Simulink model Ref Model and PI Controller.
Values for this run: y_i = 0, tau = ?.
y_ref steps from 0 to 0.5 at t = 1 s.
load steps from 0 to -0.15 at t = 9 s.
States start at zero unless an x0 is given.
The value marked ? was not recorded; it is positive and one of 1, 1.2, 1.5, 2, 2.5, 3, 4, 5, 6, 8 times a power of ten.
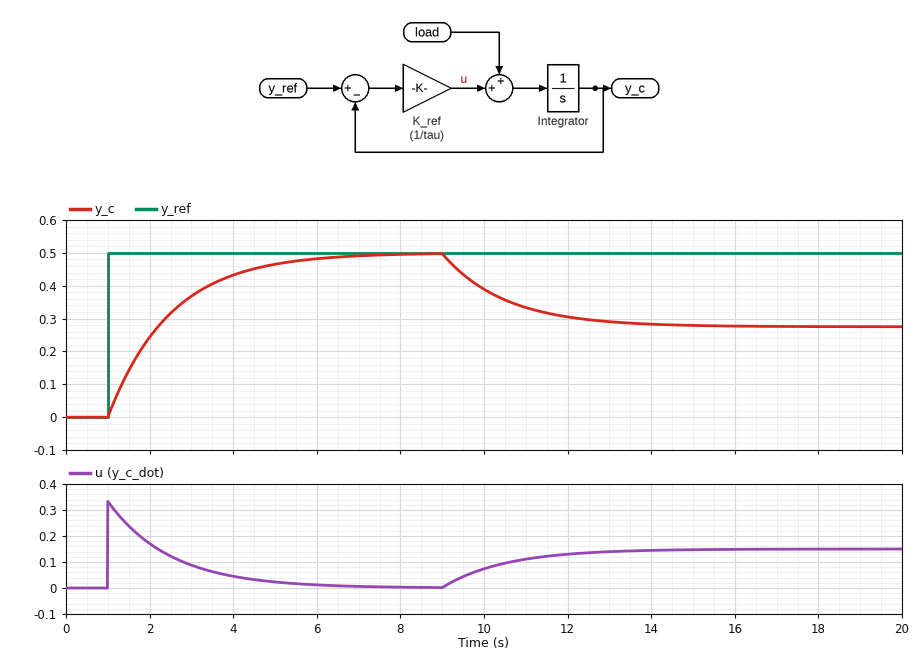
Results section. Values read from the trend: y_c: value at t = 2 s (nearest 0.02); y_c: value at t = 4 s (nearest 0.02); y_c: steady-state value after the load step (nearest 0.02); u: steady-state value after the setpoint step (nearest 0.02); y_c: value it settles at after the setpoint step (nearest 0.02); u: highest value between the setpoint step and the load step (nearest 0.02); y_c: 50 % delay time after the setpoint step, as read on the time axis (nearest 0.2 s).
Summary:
0.24
0.44
0.28
0.00
0.50
0.34
2.0 s
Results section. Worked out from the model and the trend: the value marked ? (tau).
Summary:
1.5
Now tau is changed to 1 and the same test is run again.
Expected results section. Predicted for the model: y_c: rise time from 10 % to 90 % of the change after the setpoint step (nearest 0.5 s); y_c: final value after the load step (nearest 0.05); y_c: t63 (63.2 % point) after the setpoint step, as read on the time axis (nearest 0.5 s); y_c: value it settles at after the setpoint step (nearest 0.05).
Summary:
2.0 s
0.35
2.0 s
0.50
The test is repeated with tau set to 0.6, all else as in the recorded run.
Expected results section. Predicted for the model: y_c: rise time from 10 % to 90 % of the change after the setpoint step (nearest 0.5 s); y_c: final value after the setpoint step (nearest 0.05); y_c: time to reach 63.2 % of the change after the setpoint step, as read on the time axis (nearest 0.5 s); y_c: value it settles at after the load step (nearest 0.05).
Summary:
1.5 s
0.50
1.5 s
0.40
